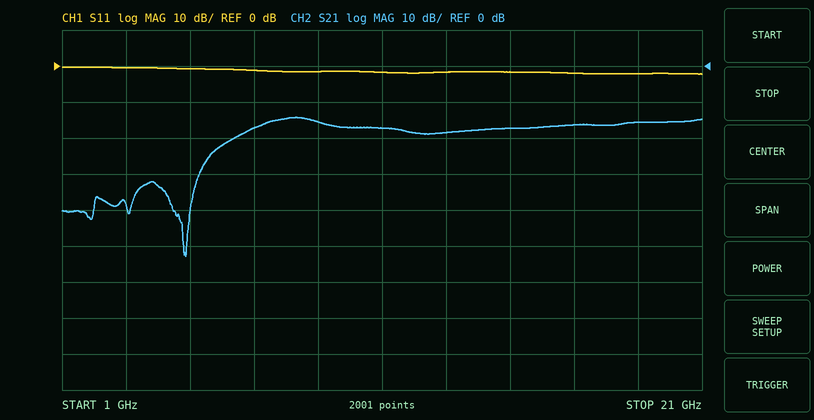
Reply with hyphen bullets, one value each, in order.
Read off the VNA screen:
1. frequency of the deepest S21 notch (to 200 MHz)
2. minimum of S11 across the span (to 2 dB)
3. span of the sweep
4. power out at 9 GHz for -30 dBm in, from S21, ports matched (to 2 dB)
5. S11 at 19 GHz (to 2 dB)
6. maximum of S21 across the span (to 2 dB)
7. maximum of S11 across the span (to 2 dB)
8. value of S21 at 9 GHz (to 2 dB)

- 4.8 GHz
- -2 dB
- 20 GHz
- -46 dBm
- -2 dB
- -14 dB
- 0 dB
- -16 dB
